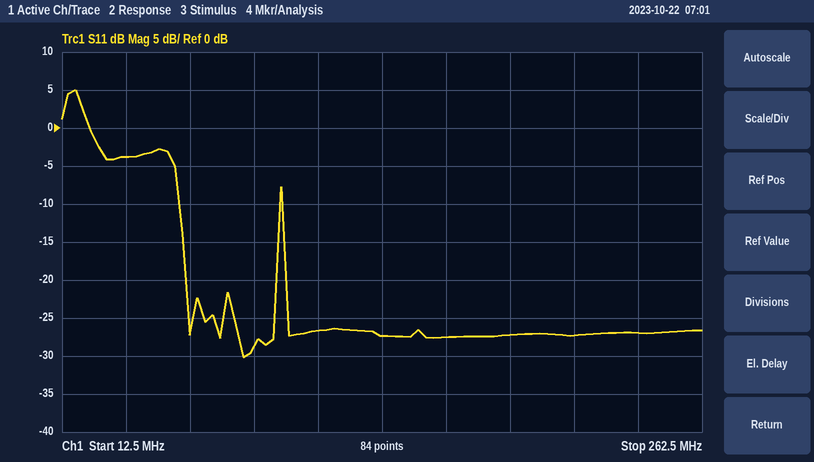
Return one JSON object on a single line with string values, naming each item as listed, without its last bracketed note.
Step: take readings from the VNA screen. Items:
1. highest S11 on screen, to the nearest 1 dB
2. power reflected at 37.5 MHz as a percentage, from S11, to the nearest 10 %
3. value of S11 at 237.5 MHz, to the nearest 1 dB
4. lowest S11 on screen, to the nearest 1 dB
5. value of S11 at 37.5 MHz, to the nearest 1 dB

{"highest S11 on screen, to the nearest 1 dB": "5 dB", "power reflected at 37.5 MHz as a percentage, from S11, to the nearest 10 %": "40 %", "value of S11 at 237.5 MHz, to the nearest 1 dB": "-27 dB", "lowest S11 on screen, to the nearest 1 dB": "-30 dB", "value of S11 at 37.5 MHz, to the nearest 1 dB": "-4 dB"}
